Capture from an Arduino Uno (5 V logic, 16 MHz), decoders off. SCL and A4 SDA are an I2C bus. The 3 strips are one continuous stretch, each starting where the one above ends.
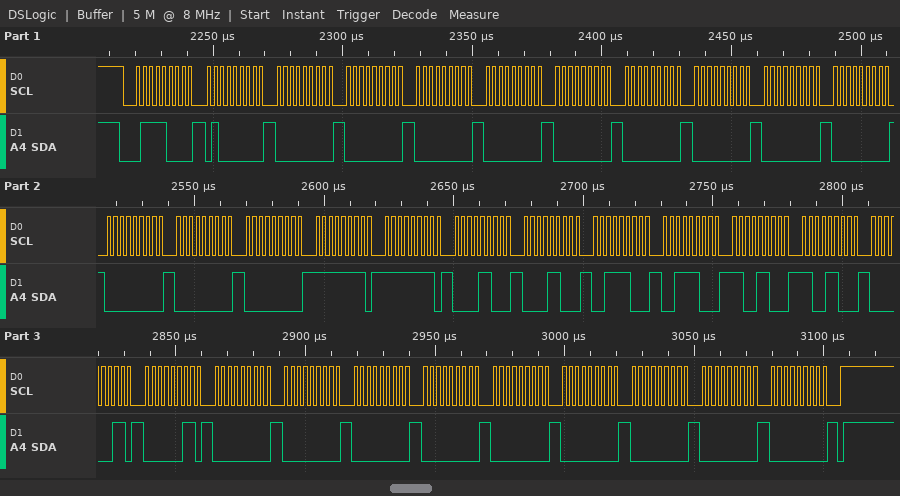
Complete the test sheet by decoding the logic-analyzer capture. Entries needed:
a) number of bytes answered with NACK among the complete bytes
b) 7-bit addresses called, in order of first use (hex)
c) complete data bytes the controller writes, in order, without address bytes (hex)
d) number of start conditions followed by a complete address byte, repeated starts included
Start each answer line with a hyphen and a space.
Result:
- 0
- 0x3C
- 40 00 00 00 00 00 00 00 00 00 00 00 00 FF FF 0C 0C 3C 3C CC CC 03 03 00 00 00 00 00 00 00 00 00
- 1
